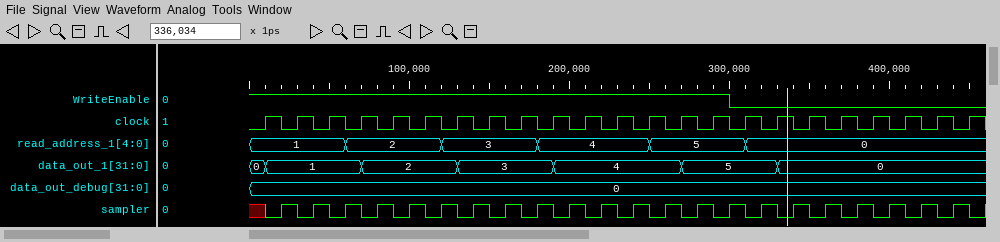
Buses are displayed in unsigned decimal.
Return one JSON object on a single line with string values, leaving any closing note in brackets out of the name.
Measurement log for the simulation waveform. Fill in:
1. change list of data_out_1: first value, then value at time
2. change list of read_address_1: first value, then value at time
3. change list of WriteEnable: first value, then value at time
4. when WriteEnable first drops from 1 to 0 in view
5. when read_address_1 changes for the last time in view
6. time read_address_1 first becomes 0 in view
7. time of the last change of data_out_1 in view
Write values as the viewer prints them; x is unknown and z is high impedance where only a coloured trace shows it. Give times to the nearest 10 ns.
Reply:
{"change list of data_out_1: first value, then value at time": "0, 1 at 10 ns, 2 at 70 ns, 3 at 130 ns, 4 at 190 ns, 5 at 270 ns, 0 at 330 ns", "change list of read_address_1: first value, then value at time": "1, 2 at 60 ns, 3 at 120 ns, 4 at 180 ns, 5 at 250 ns, 0 at 310 ns", "change list of WriteEnable: first value, then value at time": "1, 0 at 300 ns", "when WriteEnable first drops from 1 to 0 in view": "300 ns", "when read_address_1 changes for the last time in view": "310 ns", "time read_address_1 first becomes 0 in view": "310 ns", "time of the last change of data_out_1 in view": "330 ns"}
